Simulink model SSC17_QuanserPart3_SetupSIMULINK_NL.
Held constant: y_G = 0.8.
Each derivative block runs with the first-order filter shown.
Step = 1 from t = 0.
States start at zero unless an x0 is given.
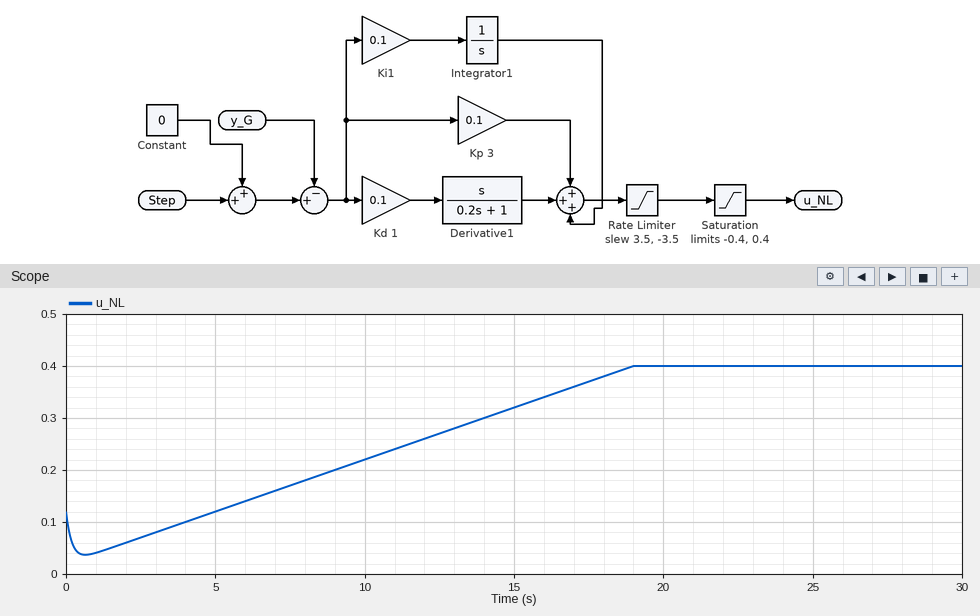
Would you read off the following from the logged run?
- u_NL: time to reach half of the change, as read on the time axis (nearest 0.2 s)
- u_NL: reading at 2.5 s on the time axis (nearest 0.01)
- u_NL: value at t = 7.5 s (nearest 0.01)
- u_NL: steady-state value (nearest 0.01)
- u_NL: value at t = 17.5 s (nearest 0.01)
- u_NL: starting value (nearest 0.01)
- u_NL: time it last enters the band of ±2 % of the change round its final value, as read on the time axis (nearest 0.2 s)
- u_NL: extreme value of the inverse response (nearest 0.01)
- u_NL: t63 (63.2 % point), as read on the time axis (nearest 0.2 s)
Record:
12.0 s
0.07
0.17
0.40
0.37
0.12
18.8 s
0.04
13.8 s
